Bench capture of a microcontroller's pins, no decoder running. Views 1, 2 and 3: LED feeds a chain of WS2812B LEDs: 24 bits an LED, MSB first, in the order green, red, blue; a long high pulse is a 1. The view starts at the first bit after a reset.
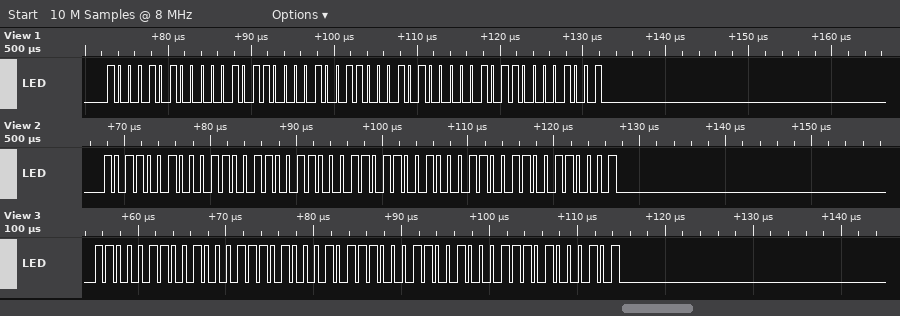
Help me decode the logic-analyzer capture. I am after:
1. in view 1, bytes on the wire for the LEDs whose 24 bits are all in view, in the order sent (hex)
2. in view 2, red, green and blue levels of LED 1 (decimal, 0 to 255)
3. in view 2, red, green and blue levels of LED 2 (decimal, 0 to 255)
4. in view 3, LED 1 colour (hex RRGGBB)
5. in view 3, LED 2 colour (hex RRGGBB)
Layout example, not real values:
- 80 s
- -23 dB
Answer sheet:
- 8A 0B 09 8A 0B 09
- 51, 178, 49
- 51, 178, 49
- #47C645
- #47C645
